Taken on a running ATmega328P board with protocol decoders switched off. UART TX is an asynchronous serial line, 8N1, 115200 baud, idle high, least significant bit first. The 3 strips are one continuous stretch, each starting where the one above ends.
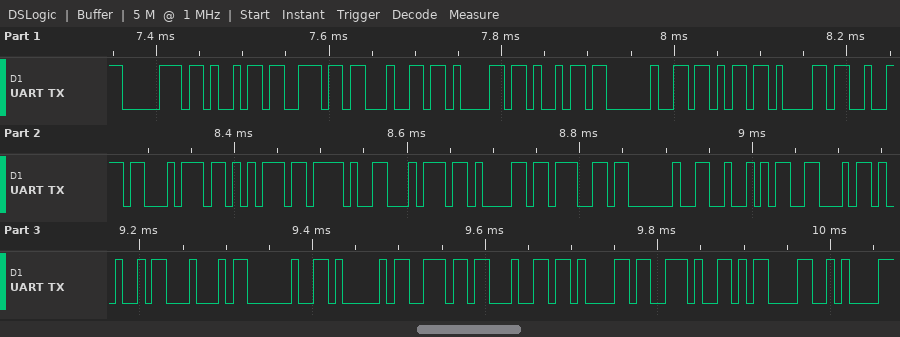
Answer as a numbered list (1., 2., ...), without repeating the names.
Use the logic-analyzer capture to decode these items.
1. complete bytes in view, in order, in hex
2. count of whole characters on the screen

1. 0x70 0x69 0x6E 0x64 0x61 0x69 0x20 0x6B 0x61 0x72 0x74 0x75 0x2F 0x74 0x61 0x67 0x20 0x52 0x46 0x49 0x44 0x20 0x41 0x6E 0x64 0x61 0x2E 0x0D 0x0A
2. 29
